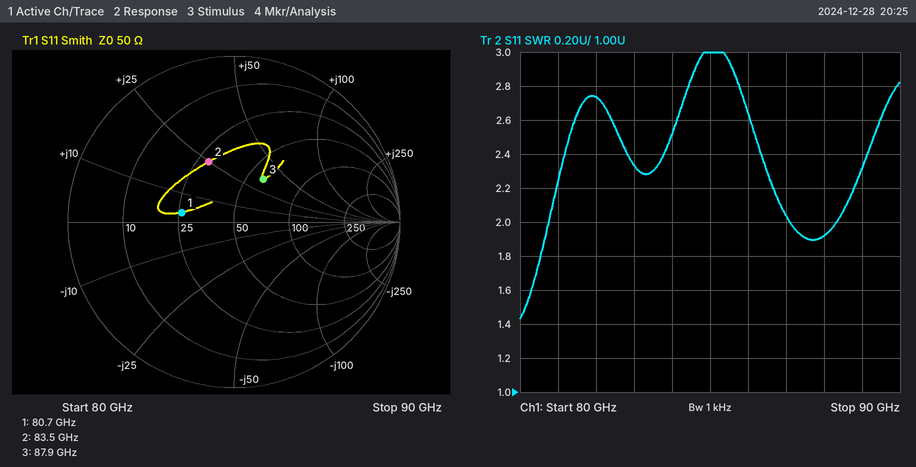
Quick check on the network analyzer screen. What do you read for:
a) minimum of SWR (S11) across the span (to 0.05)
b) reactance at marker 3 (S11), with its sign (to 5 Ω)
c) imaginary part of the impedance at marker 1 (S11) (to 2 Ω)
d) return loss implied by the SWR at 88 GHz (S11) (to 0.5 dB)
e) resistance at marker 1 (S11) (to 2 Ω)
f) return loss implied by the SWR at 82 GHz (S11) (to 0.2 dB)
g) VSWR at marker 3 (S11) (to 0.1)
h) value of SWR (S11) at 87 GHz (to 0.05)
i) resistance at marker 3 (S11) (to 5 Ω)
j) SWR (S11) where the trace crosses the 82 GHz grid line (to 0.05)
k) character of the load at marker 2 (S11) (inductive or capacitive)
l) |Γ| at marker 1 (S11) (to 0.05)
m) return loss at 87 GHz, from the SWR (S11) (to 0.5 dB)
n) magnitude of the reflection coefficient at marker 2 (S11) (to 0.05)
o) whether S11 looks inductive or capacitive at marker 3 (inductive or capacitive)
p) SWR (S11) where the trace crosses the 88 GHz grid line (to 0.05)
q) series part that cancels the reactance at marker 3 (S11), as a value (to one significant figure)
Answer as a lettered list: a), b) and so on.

a) 1.45
b) +35 Ω
c) +4 Ω
d) 10.0 dB
e) 26 Ω
f) 6.6 dB
g) 1.9
h) 2.05
i) 60 Ω
j) 2.75
k) inductive
l) 0.30
m) 9.5 dB
n) 0.40
o) inductive
p) 1.90
q) 50 fF
